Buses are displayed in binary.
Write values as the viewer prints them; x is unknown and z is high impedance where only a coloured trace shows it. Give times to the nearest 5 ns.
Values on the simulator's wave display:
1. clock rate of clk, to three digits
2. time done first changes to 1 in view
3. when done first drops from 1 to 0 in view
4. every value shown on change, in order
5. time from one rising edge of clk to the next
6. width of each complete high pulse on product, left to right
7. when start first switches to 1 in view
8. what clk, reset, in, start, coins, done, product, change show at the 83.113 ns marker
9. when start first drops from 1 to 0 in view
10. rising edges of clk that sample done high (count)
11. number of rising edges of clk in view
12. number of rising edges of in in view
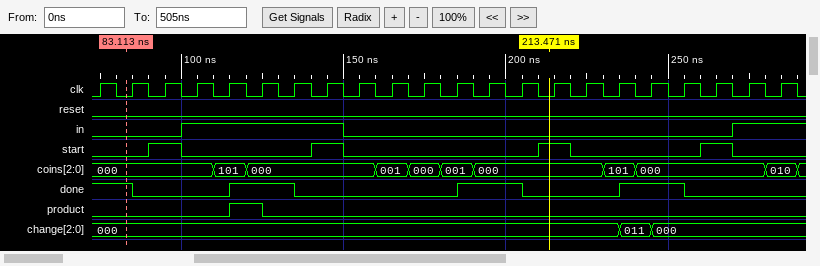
100 MHz
115 ns
85 ns
000, 011, 000
10 ns
10 ns
90 ns
clk=0, reset=0, in=0, start=0, coins=000, done=1, product=0, change=000
100 ns
8
22
2
